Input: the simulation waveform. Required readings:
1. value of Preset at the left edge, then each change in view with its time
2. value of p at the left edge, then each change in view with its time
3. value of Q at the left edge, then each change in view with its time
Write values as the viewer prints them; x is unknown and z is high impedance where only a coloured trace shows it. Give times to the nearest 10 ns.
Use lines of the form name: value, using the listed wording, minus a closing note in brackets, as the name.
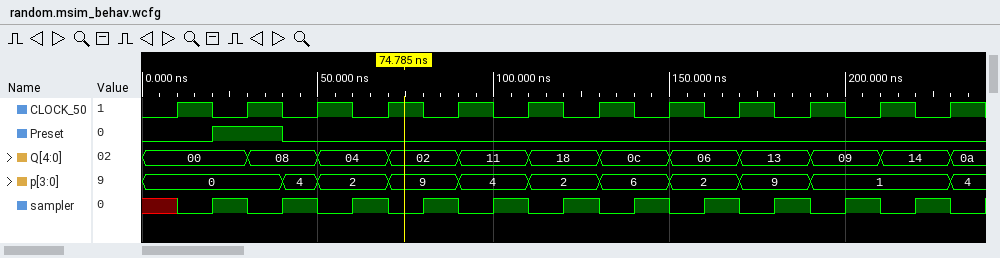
value of Preset at the left edge, then each change in view with its time: 0, 1 at 20 ns, 0 at 40 ns
value of p at the left edge, then each change in view with its time: 0, 4 at 40 ns, 2 at 50 ns, 9 at 70 ns, 4 at 90 ns, 2 at 110 ns, 6 at 130 ns, 2 at 150 ns, 9 at 170 ns, 1 at 190 ns, 4 at 230 ns
value of Q at the left edge, then each change in view with its time: 00, 08 at 30 ns, 04 at 50 ns, 02 at 70 ns, 11 at 90 ns, 18 at 110 ns, 0c at 130 ns, 06 at 150 ns, 13 at 170 ns, 09 at 190 ns, 14 at 210 ns, 0a at 230 ns
